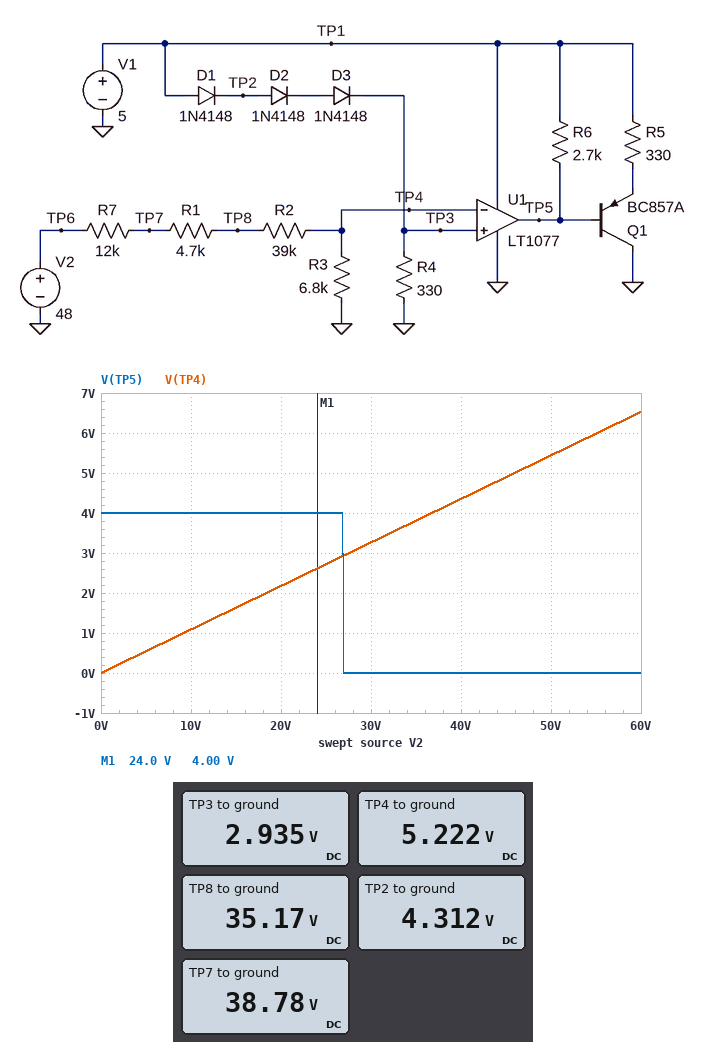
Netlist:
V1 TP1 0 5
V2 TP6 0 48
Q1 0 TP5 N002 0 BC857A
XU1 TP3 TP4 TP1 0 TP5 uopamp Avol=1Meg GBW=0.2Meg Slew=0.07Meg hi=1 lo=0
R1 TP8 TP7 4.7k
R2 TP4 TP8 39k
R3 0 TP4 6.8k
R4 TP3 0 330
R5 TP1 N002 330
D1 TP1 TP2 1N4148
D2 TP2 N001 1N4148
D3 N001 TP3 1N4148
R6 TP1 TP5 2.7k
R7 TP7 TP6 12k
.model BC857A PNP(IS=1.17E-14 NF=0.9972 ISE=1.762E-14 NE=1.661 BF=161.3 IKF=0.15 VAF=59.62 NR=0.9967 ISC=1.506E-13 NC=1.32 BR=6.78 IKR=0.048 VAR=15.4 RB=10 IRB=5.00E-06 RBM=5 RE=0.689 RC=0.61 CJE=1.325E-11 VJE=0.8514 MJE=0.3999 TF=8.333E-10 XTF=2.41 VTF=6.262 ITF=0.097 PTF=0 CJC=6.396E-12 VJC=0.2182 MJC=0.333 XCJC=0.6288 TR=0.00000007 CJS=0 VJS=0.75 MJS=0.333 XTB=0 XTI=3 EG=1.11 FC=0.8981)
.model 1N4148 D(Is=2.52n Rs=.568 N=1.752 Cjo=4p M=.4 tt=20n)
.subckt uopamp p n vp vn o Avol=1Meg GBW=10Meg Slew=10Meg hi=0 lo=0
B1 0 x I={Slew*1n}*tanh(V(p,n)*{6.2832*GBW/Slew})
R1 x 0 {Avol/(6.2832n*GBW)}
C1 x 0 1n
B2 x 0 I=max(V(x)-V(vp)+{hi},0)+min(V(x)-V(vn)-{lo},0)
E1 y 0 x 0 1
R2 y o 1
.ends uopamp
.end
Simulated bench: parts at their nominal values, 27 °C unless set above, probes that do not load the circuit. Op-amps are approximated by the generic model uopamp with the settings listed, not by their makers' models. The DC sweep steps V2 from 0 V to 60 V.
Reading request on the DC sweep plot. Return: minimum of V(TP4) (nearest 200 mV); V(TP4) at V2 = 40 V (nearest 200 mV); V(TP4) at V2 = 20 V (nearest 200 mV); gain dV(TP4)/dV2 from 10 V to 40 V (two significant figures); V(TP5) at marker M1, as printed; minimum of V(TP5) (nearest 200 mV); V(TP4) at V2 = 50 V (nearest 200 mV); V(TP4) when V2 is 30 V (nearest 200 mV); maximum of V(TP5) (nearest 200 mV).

0 V
4.4 V
2.2 V
0.11 V/V
4.00 V
0 V
5.4 V
3.2 V
4.0 V
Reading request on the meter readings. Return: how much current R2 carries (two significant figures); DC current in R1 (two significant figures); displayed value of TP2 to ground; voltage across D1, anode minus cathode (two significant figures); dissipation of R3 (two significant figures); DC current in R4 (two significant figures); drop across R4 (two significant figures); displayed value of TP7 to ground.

770 µA
770 µA
4.312 V
690 mV
4.0 mW
8.9 mA
2.9 V
38.78 V
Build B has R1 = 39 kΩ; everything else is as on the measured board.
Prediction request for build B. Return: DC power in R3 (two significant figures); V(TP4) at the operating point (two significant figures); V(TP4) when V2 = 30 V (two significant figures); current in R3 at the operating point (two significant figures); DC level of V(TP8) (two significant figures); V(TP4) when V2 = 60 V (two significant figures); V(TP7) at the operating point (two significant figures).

1.7 mW
3.4 V
2.1 V
500 µA
23 V
4.2 V
42 V
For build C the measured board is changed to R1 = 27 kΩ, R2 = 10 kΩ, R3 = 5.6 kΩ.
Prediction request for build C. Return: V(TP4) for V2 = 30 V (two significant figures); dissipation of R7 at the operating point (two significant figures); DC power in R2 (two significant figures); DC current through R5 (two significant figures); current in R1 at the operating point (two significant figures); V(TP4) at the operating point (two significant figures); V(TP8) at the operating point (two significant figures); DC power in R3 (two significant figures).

3.1 V
9.3 mW
7.7 mW
13 mA
880 µA
4.9 V
14 V
4.3 mW
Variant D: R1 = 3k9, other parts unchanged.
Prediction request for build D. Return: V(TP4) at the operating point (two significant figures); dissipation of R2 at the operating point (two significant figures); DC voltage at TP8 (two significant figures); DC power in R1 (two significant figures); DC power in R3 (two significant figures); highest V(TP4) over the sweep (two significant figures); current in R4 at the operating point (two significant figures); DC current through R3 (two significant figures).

5.3 V
24 mW
36 V
2.4 mW
4.1 mW
6.6 V
8.9 mA
780 µA
